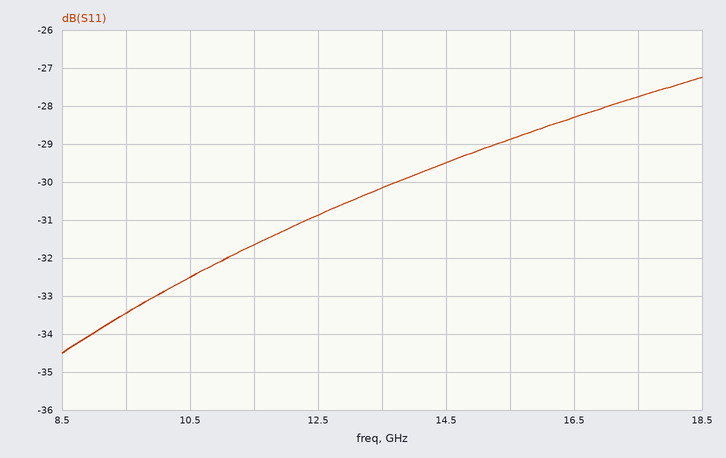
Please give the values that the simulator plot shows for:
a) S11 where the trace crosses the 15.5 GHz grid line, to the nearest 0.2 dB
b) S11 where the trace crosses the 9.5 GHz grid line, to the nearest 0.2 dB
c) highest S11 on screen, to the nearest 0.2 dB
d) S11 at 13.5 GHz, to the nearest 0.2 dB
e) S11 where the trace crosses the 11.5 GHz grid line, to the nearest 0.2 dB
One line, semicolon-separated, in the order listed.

-28.8 dB; -33.4 dB; -27.2 dB; -30.2 dB; -31.6 dB
